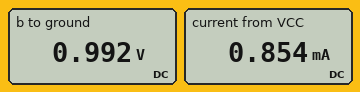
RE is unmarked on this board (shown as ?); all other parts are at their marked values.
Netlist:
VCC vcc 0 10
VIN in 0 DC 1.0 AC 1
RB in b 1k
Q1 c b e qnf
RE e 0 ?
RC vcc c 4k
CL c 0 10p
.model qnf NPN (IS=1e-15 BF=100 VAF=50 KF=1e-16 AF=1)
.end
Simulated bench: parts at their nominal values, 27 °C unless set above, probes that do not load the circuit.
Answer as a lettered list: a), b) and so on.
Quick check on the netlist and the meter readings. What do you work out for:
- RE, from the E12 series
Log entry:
a) 330 Ω
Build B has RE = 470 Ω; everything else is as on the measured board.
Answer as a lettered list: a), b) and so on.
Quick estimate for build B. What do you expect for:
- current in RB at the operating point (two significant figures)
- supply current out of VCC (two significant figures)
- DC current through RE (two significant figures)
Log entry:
a) 5.5 µA
b) 620 µA
c) 630 µA
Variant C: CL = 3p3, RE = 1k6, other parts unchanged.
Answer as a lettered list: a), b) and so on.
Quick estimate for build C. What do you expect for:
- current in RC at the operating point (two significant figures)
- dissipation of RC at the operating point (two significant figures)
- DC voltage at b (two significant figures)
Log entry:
a) 200 µA
b) 170 µW
c) 1.0 V
